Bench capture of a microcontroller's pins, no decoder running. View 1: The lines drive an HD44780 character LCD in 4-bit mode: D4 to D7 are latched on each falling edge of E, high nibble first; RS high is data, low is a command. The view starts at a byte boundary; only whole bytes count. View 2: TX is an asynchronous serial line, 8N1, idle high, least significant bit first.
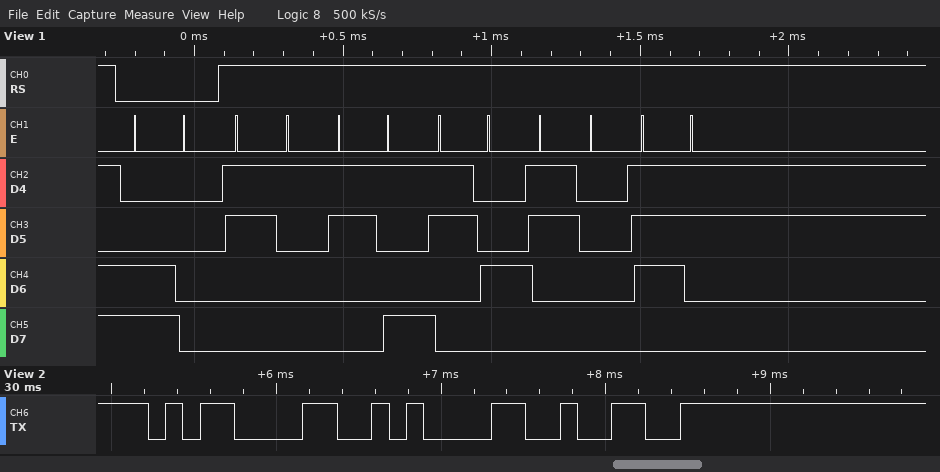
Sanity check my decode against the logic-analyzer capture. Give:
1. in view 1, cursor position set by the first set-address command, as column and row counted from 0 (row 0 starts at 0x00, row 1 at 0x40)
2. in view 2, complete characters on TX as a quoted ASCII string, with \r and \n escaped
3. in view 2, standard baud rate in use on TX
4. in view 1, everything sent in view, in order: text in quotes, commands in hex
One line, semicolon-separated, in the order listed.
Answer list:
column 0, row 1; "\r\n2"; 9600 baud; 0xC0 "1940s"
